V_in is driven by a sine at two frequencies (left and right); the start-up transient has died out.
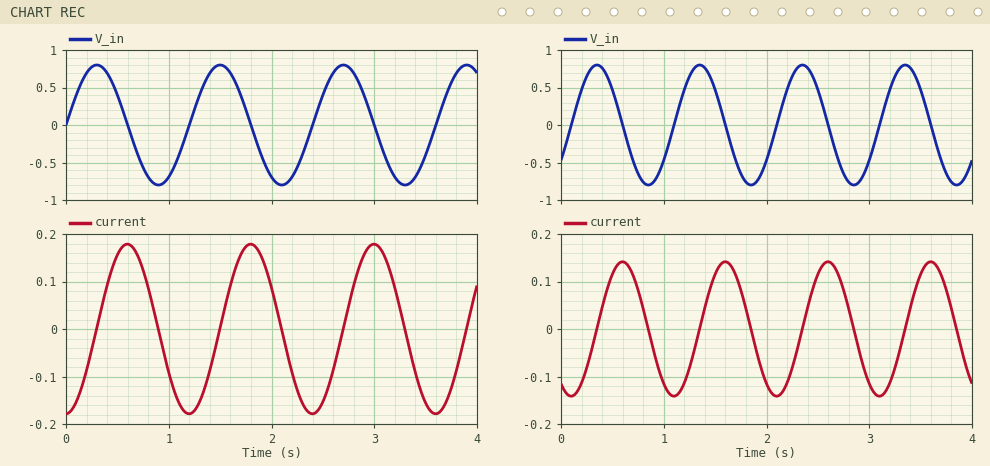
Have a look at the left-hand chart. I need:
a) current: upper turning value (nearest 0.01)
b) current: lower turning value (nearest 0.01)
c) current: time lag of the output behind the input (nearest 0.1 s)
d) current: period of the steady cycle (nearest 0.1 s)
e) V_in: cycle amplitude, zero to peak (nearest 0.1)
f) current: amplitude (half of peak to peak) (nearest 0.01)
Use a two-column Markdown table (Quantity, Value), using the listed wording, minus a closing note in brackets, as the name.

| Quantity | Value |
|---|---|
| current: upper turning value | 0.18 |
| current: lower turning value | -0.18 |
| current: time lag of the output behind the input | 0.3 s |
| current: period of the steady cycle | 1.2 s |
| V_in: cycle amplitude, zero to peak | 0.8 |
| current: amplitude (half of peak to peak) | 0.18 |
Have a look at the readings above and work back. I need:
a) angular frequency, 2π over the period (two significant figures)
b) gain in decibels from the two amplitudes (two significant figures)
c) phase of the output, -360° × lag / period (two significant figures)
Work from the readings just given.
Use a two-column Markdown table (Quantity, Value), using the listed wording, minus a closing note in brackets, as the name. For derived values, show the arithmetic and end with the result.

| Quantity | Value |
|---|---|
| angular frequency, 2π over the period | 2π / 1.2 = 5.2 rad/s |
| gain in decibels from the two amplitudes | 20 log10(0.18 / 0.8) = -13 dB |
| phase of the output, -360° × lag / period | -360 × 0.3 / 1.2 = -90° |
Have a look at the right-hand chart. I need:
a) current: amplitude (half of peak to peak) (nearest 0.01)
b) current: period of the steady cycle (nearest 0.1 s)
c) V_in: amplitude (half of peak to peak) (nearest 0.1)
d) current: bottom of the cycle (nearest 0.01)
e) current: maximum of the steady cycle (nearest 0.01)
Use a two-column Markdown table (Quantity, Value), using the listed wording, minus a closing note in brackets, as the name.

| Quantity | Value |
|---|---|
| current: amplitude (half of peak to peak) | 0.14 |
| current: period of the steady cycle | 1.0 s |
| V_in: amplitude (half of peak to peak) | 0.8 |
| current: bottom of the cycle | -0.14 |
| current: maximum of the steady cycle | 0.14 |
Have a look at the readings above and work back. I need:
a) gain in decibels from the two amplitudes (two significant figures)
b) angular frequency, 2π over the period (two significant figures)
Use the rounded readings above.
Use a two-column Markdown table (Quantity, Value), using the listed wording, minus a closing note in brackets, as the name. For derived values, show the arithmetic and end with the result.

| Quantity | Value |
|---|---|
| gain in decibels from the two amplitudes | 20 log10(0.14 / 0.8) = -15 dB |
| angular frequency, 2π over the period | 2π / 1 = 6.3 rad/s |
